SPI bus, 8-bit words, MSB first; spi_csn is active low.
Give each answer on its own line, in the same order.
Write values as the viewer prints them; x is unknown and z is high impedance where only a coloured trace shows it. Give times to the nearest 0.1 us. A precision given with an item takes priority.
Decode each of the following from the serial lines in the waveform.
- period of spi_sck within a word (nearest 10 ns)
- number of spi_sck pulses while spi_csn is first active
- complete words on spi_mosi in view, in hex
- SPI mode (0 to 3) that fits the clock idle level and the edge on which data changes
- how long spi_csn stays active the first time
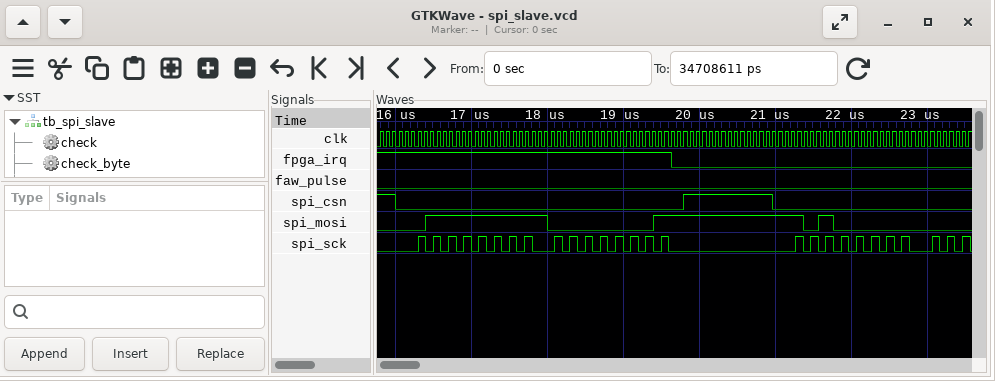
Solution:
200 ns
16
7F, 01, A0
0
3.8 us
